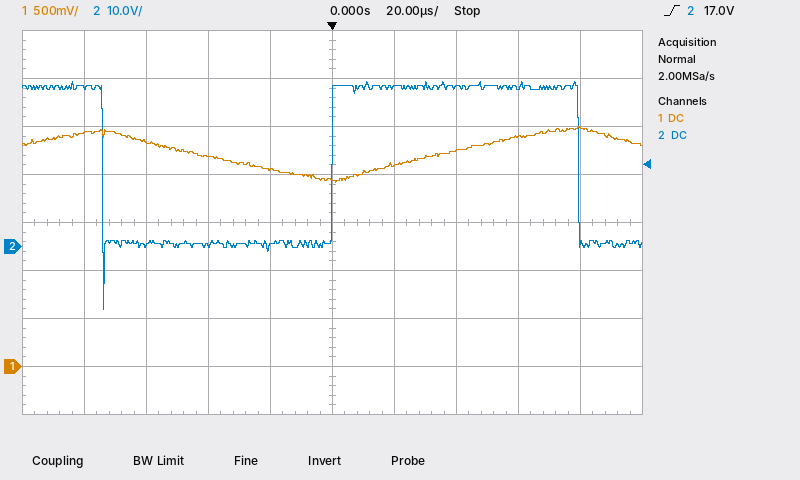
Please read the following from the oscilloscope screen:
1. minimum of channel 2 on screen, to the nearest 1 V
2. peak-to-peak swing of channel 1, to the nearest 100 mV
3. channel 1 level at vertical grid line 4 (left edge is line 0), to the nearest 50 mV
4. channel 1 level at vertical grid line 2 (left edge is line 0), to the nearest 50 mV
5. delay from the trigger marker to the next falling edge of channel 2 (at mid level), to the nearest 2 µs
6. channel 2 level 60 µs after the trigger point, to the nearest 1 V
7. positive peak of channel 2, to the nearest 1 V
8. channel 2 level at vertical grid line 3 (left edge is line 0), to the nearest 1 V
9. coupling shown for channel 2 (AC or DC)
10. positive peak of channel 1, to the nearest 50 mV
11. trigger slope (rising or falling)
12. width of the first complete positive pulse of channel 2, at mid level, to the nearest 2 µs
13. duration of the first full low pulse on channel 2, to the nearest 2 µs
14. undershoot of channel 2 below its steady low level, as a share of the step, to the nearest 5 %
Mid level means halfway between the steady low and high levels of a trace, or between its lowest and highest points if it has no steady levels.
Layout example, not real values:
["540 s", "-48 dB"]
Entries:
["-13 V", "600 mV", "2.05 V", "2.35 V", "80 µs", "33 V", "34 V", "0 V", "DC", "2.50 V", "rising", "80 µs", "74 µs", "40 %"]
